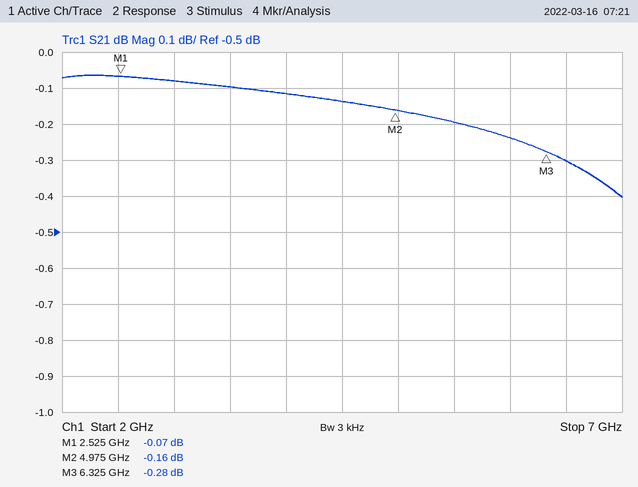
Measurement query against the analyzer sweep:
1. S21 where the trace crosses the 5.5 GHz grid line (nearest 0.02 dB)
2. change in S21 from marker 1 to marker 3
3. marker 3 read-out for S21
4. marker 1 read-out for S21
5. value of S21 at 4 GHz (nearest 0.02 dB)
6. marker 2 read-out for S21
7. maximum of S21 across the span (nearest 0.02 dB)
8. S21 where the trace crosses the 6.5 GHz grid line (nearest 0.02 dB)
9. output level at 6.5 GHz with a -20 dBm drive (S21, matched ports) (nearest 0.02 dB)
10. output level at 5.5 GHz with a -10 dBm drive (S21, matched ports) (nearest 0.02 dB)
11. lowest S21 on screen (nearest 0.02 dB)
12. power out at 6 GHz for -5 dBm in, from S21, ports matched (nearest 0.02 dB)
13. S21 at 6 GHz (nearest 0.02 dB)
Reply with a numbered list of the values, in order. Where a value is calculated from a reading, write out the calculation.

1. -0.20 dB
2. -0.28 − (-0.07) = -0.21 dB
3. -0.28 dB
4. -0.07 dB
5. -0.12 dB
6. -0.16 dB
7. -0.06 dB
8. -0.30 dB
9. -20 dBm + (-0.30 dB) = -20.30 dBm
10. -10 dBm + (-0.20 dB) = -10.20 dBm
11. -0.40 dB
12. -5 dBm + (-0.24 dB) = -5.24 dBm
13. -0.24 dB
